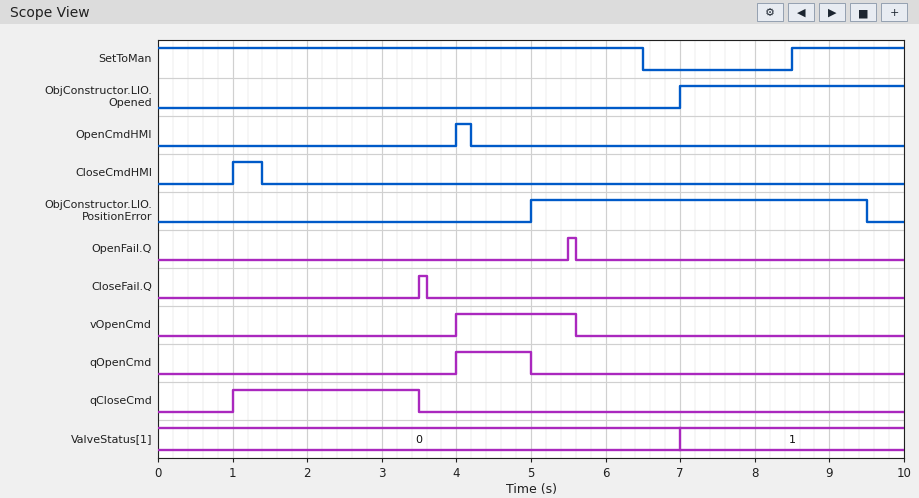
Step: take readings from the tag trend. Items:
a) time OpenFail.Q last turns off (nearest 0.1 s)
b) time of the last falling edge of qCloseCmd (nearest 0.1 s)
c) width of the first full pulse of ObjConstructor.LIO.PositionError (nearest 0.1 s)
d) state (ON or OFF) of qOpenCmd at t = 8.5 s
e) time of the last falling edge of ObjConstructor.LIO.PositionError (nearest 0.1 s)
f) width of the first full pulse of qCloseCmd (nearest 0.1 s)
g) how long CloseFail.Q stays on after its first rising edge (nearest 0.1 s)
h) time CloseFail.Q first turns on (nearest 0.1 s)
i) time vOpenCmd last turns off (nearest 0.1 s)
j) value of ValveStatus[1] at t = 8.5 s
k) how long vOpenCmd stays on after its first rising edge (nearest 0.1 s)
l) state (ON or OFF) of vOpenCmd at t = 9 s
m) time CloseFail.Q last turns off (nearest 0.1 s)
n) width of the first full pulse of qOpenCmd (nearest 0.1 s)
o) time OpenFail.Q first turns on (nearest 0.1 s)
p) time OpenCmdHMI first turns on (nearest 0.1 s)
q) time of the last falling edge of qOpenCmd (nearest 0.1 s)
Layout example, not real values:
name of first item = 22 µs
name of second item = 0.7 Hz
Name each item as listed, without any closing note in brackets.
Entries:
time OpenFail.Q last turns off = 5.6 s
time of the last falling edge of qCloseCmd = 3.5 s
width of the first full pulse of ObjConstructor.LIO.PositionError = 4.5 s
state (ON or OFF) of qOpenCmd at t = 8.5 s = OFF
time of the last falling edge of ObjConstructor.LIO.PositionError = 9.5 s
width of the first full pulse of qCloseCmd = 2.5 s
how long CloseFail.Q stays on after its first rising edge = 0.1 s
time CloseFail.Q first turns on = 3.5 s
time vOpenCmd last turns off = 5.6 s
value of ValveStatus[1] at t = 8.5 s = 1
how long vOpenCmd stays on after its first rising edge = 1.6 s
state (ON or OFF) of vOpenCmd at t = 9 s = OFF
time CloseFail.Q last turns off = 3.6 s
width of the first full pulse of qOpenCmd = 1.0 s
time OpenFail.Q first turns on = 5.5 s
time OpenCmdHMI first turns on = 4.0 s
time of the last falling edge of qOpenCmd = 5.0 s
